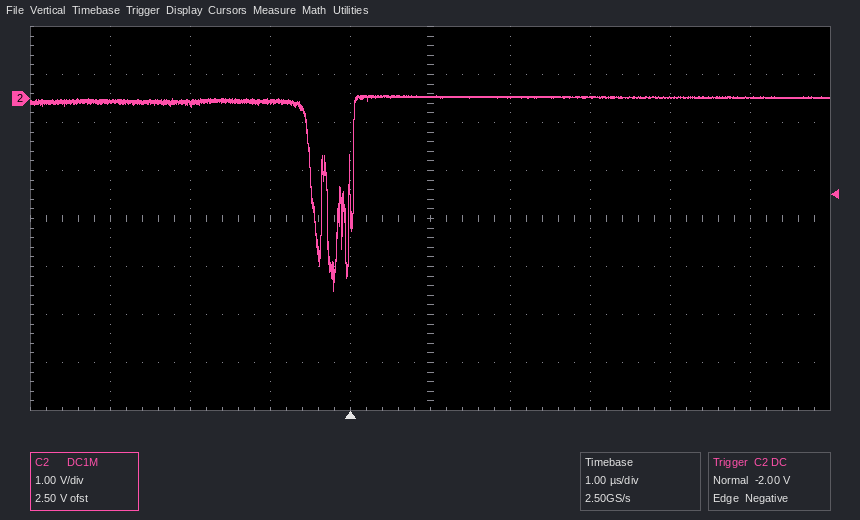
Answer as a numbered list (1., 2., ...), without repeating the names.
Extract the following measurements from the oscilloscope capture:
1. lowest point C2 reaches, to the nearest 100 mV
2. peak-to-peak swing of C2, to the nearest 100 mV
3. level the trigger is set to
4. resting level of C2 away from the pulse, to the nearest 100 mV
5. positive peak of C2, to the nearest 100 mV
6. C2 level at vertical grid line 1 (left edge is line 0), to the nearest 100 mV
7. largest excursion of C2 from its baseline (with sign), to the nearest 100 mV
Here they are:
1. -4.0 V
2. 4.1 V
3. -2.00 V
4. 0.0 V
5. 100 mV
6. -100 mV
7. -4.0 V
